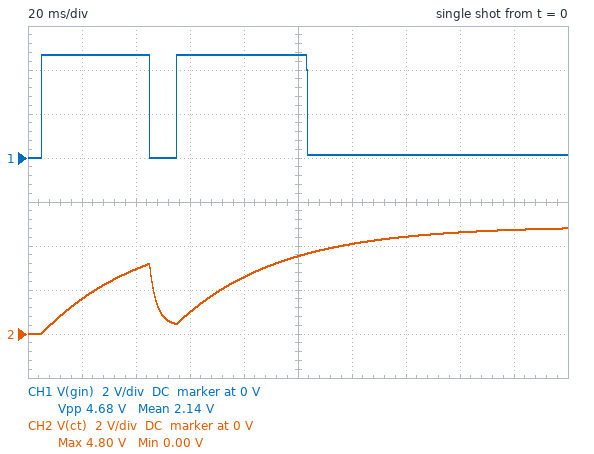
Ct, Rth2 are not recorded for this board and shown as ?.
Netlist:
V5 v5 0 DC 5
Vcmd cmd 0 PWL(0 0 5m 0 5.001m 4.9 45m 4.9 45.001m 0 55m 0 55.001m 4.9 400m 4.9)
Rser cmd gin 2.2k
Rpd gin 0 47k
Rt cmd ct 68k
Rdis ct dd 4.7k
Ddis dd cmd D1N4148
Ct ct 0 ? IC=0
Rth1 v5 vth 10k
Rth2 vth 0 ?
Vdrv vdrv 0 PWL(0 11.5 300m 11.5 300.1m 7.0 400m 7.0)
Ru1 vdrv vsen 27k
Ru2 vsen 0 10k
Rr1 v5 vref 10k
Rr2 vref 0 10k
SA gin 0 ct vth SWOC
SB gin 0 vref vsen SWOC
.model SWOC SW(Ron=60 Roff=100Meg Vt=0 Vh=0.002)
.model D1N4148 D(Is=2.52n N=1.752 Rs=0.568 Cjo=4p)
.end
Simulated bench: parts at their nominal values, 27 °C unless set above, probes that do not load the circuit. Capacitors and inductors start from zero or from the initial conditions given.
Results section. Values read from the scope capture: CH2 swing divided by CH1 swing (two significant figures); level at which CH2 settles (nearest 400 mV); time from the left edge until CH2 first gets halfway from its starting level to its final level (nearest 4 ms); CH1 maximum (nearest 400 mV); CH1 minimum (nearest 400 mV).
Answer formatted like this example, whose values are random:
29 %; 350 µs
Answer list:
1.0; 4.8 V; 32 ms; 4.8 V; 0 V
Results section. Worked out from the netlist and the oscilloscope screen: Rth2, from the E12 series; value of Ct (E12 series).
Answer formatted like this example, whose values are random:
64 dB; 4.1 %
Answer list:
27 kΩ; 560 nF
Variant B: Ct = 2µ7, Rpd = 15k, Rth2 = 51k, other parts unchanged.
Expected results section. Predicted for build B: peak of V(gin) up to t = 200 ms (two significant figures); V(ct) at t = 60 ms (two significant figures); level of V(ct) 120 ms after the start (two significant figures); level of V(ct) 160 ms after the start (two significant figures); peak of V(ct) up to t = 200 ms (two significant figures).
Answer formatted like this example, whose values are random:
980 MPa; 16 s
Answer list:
4.3 V; 770 mV; 1.9 V; 2.5 V; 3.0 V
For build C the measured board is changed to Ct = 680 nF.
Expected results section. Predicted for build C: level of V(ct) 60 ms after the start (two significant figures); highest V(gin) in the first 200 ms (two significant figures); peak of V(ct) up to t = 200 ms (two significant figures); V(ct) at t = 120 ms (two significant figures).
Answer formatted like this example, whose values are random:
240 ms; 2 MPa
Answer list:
950 mV; 4.7 V; 4.7 V; 3.8 V
